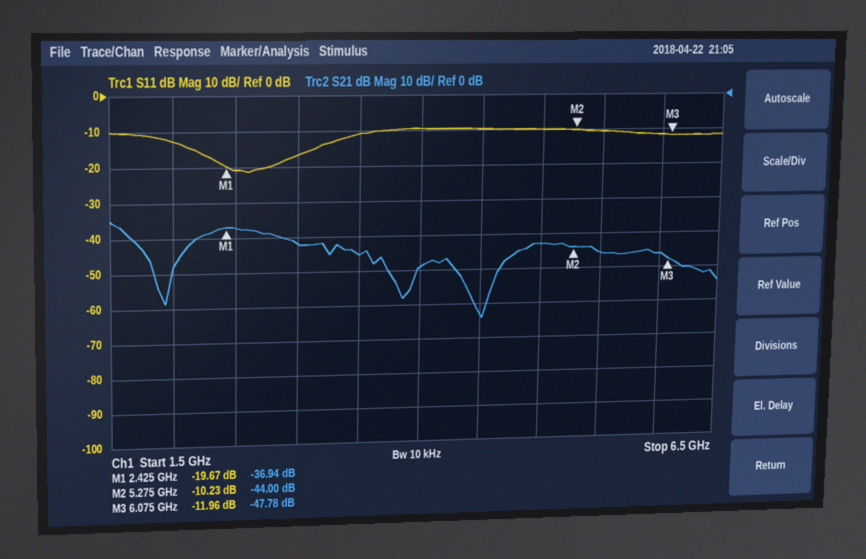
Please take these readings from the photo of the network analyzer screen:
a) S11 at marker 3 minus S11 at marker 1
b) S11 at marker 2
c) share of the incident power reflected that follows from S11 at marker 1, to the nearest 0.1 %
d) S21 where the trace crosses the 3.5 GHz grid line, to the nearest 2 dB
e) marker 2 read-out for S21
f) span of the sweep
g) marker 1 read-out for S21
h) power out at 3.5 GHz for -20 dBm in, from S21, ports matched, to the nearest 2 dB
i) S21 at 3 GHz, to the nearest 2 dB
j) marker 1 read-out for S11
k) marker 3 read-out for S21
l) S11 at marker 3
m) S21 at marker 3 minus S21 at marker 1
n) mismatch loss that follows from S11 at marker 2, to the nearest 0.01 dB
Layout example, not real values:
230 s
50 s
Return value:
7.71 dB
-10.23 dB
1.1 %
-46 dB
-44.00 dB
5 GHz
-36.94 dB
-66 dBm
-42 dB
-19.67 dB
-47.78 dB
-11.96 dB
-10.84 dB
0.43 dB
